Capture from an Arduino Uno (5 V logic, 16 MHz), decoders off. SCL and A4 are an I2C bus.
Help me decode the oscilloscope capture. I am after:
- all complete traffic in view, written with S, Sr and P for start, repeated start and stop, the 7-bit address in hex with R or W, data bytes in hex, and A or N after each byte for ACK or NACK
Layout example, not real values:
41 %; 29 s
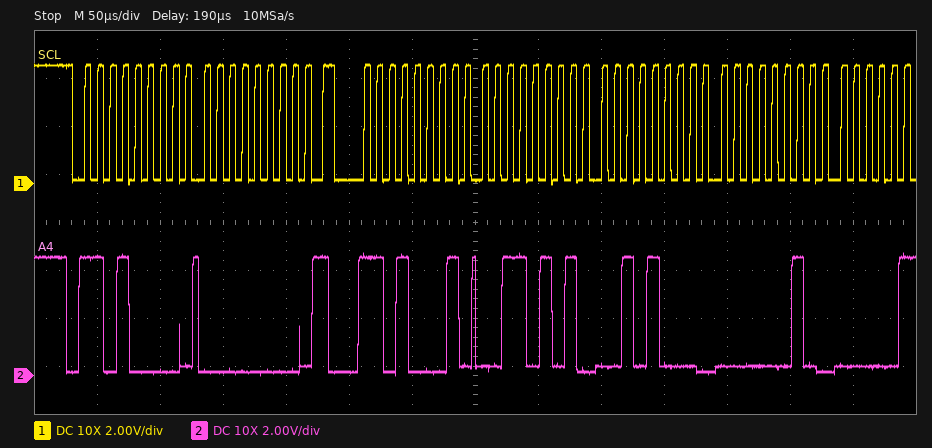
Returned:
S 68W A 00 A Sr 68R A 35 A 28 A 02 A
